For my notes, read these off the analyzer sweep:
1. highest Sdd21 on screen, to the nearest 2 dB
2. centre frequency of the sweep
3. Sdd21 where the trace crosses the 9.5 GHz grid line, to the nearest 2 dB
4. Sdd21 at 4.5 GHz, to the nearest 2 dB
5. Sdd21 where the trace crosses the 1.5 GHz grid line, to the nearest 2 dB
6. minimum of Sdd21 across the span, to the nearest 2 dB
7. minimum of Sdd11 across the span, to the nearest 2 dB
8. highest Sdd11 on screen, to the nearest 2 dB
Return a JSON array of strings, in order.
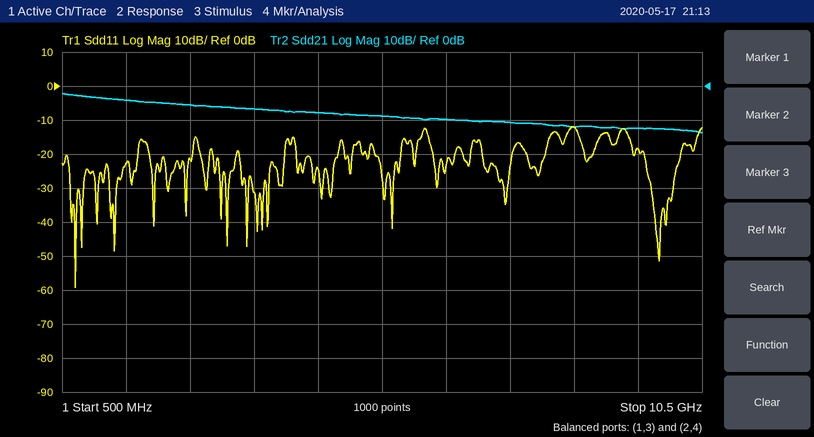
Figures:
["-2 dB", "5.5 GHz", "-12 dB", "-8 dB", "-4 dB", "-14 dB", "-60 dB", "-12 dB"]
